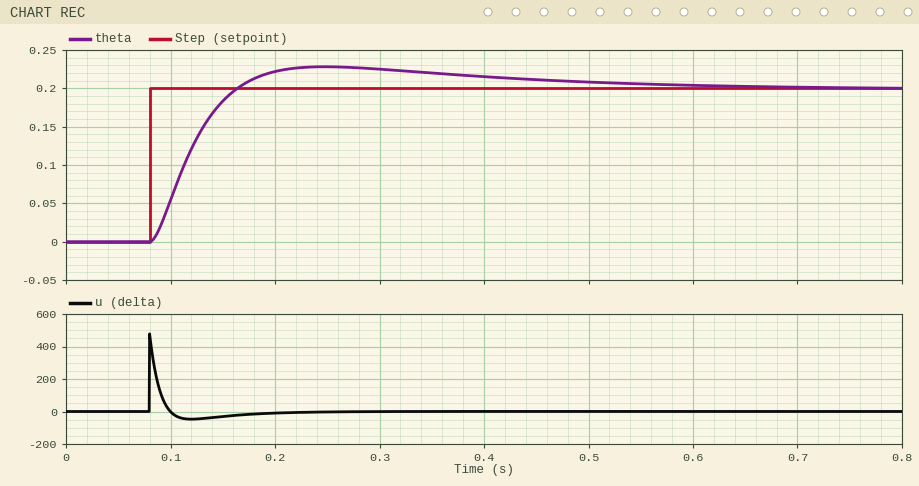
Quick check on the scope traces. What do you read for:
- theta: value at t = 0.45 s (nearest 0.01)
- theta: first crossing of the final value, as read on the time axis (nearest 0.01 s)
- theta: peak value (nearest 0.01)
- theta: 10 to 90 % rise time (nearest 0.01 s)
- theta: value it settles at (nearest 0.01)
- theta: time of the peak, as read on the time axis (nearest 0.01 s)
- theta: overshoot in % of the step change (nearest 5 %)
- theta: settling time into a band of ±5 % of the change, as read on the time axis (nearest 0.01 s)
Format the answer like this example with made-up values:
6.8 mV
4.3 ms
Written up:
0.21
0.16 s
0.23
0.06 s
0.20
0.25 s
15 %
0.47 s
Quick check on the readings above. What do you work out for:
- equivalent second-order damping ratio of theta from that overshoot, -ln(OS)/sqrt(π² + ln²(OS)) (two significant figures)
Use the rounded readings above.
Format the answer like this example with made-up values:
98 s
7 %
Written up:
0.52
